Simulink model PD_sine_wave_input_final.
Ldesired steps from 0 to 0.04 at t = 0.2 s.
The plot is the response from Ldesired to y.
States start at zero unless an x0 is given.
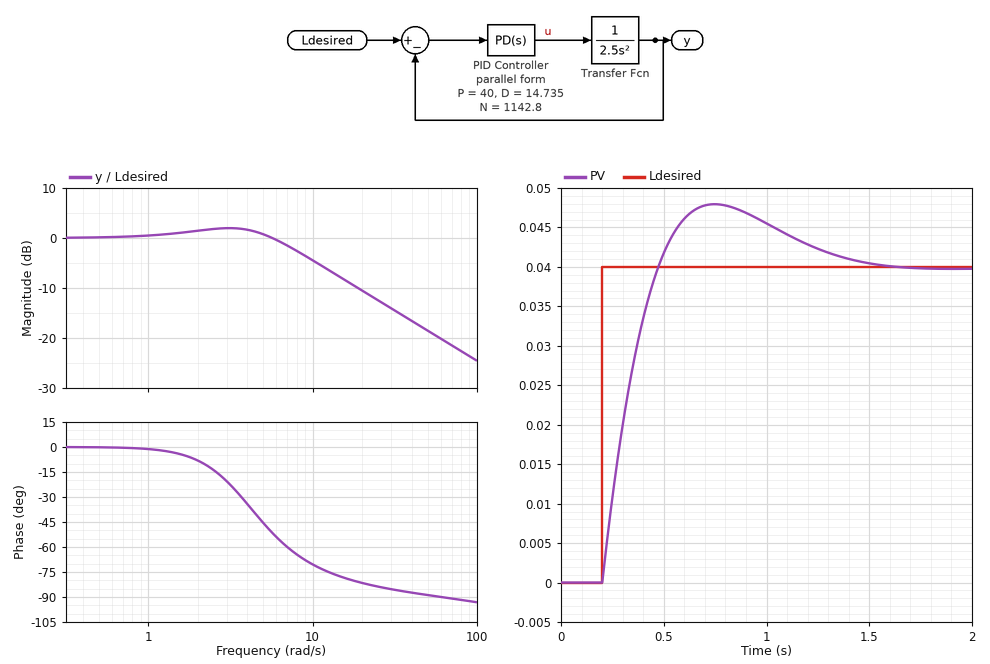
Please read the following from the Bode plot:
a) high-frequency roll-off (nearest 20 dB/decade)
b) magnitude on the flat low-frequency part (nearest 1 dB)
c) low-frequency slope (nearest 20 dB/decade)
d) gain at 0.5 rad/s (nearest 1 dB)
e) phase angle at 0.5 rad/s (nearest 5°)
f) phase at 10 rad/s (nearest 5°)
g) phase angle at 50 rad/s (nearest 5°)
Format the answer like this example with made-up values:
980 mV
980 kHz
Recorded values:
-20 dB/decade
0 dB
0 dB/decade
0 dB
0°
-70°
-90°
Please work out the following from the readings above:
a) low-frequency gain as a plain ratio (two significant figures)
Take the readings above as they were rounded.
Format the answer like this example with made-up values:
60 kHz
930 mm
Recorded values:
1.0
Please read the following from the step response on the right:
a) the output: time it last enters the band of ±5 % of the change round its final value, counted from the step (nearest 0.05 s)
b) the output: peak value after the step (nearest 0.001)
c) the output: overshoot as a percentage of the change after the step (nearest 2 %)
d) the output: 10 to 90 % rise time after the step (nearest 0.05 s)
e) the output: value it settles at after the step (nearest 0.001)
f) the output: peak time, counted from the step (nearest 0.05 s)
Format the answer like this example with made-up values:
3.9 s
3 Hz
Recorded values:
1.10 s
0.048
20 %
0.20 s
0.040
0.55 s
